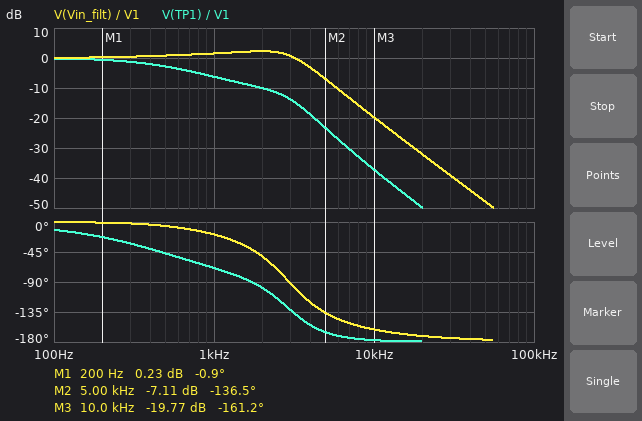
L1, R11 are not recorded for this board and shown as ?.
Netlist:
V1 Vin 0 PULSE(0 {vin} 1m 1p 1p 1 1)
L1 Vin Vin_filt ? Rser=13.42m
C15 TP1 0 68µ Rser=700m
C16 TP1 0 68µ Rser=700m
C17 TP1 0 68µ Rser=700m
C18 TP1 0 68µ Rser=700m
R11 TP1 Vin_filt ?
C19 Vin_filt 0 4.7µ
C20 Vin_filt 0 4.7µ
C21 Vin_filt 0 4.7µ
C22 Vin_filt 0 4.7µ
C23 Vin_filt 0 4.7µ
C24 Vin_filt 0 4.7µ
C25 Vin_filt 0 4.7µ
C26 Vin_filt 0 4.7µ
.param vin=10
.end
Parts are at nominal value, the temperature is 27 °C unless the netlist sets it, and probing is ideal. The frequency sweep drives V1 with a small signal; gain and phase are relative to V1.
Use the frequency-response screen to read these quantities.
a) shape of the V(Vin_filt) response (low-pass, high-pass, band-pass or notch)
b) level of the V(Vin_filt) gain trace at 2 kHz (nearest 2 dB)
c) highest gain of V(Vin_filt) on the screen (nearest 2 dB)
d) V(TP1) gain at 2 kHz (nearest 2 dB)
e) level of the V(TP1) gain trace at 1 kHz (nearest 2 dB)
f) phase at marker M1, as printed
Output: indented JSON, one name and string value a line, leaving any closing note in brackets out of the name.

{
  "shape of the V(Vin_filt) response": "low-pass",
  "level of the V(Vin_filt) gain trace at 2 kHz": "2 dB",
  "highest gain of V(Vin_filt) on the screen": "2 dB",
  "V(TP1) gain at 2 kHz": "-10 dB",
  "level of the V(TP1) gain trace at 1 kHz": "-6 dB",
  "phase at marker M1, as printed": "-0.9 deg"
}
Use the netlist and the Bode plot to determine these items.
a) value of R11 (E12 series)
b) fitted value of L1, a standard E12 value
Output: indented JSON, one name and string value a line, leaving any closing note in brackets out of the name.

{
  "value of R11": "1.2 Ω",
  "fitted value of L1, a standard E12 value": "68 µH"
}
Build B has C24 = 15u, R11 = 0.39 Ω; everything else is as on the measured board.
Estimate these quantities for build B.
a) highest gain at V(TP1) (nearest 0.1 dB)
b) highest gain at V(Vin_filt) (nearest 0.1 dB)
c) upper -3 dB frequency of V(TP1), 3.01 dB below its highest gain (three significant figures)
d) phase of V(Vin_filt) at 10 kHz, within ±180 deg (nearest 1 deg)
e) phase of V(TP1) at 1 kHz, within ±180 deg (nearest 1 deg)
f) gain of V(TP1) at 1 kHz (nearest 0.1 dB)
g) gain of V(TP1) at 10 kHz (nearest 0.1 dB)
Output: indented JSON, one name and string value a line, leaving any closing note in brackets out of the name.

{
  "highest gain at V(TP1)": "1.6 dB",
  "highest gain at V(Vin_filt)": "4.0 dB",
  "upper -3 dB frequency of V(TP1), 3.01 dB below its highest gain": "1.41 kHz",
  "phase of V(Vin_filt) at 10 kHz, within ±180 deg": "-149 deg",
  "phase of V(TP1) at 1 kHz, within ±180 deg": "-64 deg",
  "gain of V(TP1) at 1 kHz": "1.5 dB",
  "gain of V(TP1) at 10 kHz": "-33.1 dB"
}
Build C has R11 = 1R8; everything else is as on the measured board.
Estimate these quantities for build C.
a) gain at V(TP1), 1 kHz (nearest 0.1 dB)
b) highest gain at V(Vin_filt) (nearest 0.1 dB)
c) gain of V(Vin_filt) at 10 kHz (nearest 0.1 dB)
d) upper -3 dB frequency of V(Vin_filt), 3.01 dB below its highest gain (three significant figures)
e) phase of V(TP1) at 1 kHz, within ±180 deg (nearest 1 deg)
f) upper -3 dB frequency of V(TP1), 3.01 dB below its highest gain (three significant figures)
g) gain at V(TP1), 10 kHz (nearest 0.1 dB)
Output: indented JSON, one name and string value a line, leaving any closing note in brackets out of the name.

{
  "gain at V(TP1), 1 kHz": "-9.4 dB",
  "highest gain at V(Vin_filt)": "4.1 dB",
  "gain of V(Vin_filt) at 10 kHz": "-19.5 dB",
  "upper -3 dB frequency of V(Vin_filt), 3.01 dB below its highest gain": "3.62 kHz",
  "phase of V(TP1) at 1 kHz, within ±180 deg": "-70 deg",
  "upper -3 dB frequency of V(TP1), 3.01 dB below its highest gain": "324 Hz",
  "gain at V(TP1), 10 kHz": "-40.1 dB"
}
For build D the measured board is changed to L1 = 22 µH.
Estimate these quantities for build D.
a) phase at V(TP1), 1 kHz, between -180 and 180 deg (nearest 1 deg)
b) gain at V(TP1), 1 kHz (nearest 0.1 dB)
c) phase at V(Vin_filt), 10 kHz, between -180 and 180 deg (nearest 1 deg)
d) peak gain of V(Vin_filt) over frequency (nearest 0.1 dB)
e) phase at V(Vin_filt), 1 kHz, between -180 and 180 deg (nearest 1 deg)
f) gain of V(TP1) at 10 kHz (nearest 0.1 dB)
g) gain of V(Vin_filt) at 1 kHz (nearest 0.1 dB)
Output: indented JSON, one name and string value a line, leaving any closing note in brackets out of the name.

{
  "phase at V(TP1), 1 kHz, between -180 and 180 deg": "-56 deg",
  "gain at V(TP1), 1 kHz": "-7.3 dB",
  "phase at V(Vin_filt), 10 kHz, between -180 and 180 deg": "-156 deg",
  "peak gain of V(Vin_filt) over frequency": "5.4 dB",
  "phase at V(Vin_filt), 1 kHz, between -180 and 180 deg": "-6 deg",
  "gain of V(TP1) at 10 kHz": "-25.5 dB",
  "gain of V(Vin_filt) at 1 kHz": "0.5 dB"
}
